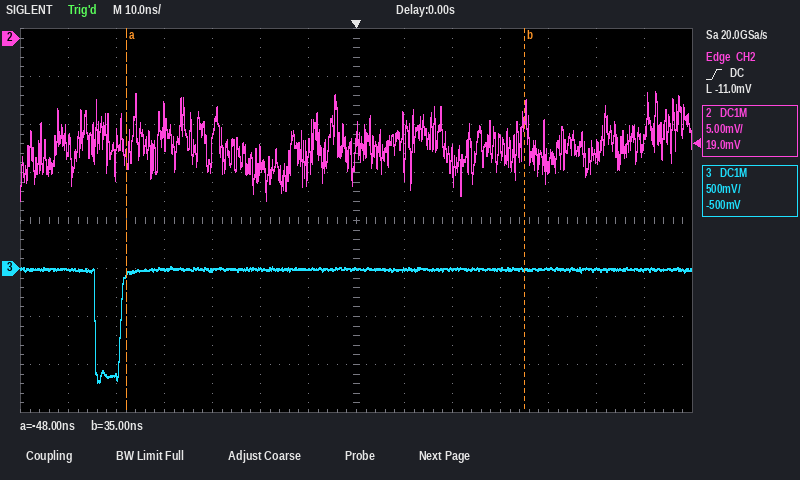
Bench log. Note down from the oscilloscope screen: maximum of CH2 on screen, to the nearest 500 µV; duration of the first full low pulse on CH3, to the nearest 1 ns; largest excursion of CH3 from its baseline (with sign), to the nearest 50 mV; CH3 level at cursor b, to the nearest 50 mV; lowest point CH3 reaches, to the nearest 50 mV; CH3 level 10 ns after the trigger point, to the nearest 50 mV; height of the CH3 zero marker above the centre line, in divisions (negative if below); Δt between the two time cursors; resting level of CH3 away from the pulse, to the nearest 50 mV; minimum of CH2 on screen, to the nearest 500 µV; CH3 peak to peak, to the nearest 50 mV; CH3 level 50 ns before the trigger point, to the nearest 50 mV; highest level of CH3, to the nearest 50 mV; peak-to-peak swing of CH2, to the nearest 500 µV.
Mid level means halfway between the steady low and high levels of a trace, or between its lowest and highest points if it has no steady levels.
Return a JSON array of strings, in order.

["-5.5 mV", "5 ns", "-1.20 V", "0 mV", "-1.20 V", "0 mV", "-1.0 div", "83 ns", "0 mV", "-17.0 mV", "1.20 V", "-1.15 V", "0 mV", "11.5 mV"]
